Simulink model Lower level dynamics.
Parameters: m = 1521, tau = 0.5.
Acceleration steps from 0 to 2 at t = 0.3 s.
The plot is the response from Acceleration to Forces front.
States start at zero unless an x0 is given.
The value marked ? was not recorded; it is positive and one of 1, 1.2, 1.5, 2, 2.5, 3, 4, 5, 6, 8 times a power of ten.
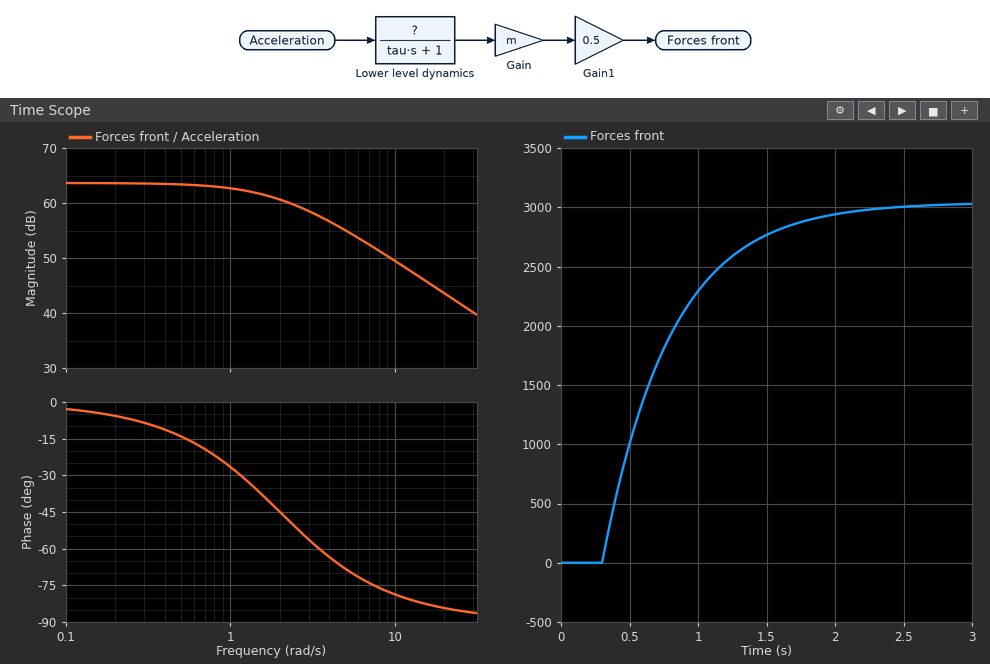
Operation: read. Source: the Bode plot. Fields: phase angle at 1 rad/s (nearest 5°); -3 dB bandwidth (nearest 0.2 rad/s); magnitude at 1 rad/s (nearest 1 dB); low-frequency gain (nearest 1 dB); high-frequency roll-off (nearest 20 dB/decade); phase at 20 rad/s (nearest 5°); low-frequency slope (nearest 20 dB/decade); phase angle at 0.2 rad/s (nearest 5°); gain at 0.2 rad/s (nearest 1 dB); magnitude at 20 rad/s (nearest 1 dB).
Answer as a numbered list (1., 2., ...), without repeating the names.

1. -25°
2. 2.0 rad/s
3. 63 dB
4. 64 dB
5. -20 dB/decade
6. -85°
7. 0 dB/decade
8. -5°
9. 64 dB
10. 44 dB
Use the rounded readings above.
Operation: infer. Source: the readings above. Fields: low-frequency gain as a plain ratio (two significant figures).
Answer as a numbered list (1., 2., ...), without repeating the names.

1. 1600
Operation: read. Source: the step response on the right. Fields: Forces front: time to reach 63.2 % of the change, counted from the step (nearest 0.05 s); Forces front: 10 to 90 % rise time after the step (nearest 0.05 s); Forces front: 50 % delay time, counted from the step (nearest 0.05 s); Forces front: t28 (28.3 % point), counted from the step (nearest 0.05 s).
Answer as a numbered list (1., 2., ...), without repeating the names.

1. 0.50 s
2. 1.10 s
3. 0.35 s
4. 0.15 s
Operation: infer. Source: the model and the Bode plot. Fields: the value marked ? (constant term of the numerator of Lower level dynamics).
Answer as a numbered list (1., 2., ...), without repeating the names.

1. 2
